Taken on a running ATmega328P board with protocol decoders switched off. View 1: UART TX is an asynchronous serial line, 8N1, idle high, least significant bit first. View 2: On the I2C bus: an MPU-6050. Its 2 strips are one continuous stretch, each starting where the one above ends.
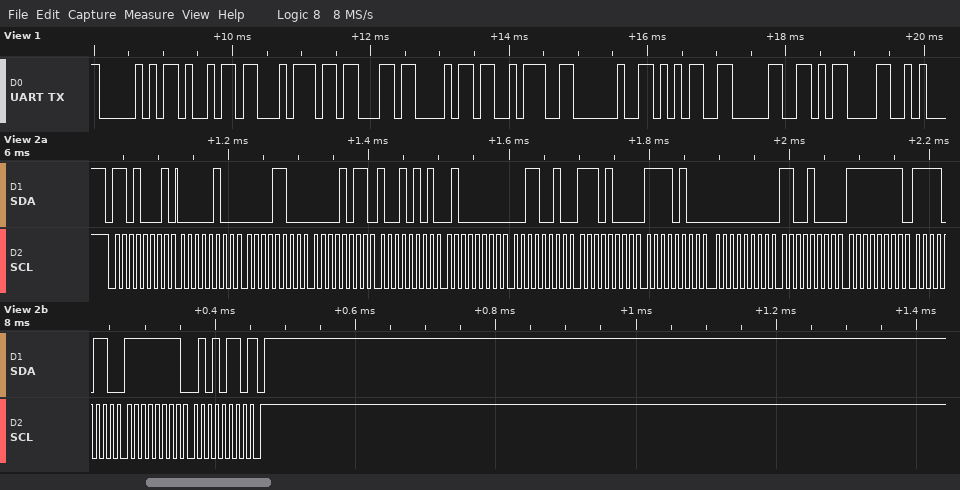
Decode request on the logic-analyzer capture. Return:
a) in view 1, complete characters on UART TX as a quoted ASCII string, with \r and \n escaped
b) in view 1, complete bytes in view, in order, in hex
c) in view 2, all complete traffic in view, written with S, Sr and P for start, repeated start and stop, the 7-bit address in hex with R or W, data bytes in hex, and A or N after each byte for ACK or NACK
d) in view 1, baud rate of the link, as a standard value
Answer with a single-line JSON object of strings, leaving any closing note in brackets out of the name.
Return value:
{"in view 1, complete characters on UART TX as a quoted ASCII string, with \\r and \\n escaped": "\"Pitch: 50\\r\"", "in view 1, complete bytes in view, in order, in hex": "50 69 74 63 68 3A 20 35 30 0D", "in view 2, all complete traffic in view, written with S, Sr and P for start, repeated start and stop, the 7-bit address in hex with R or W, data bytes in hex, and A or N after each byte for ACK or NACK": "S 68R A 04 A 0C A 0B A 95 A 40 A 32 A E8 A F4 A 00 A C8 A FF A F6 A FF A 56 N P", "in view 1, baud rate of the link, as a standard value": "9600 baud"}
